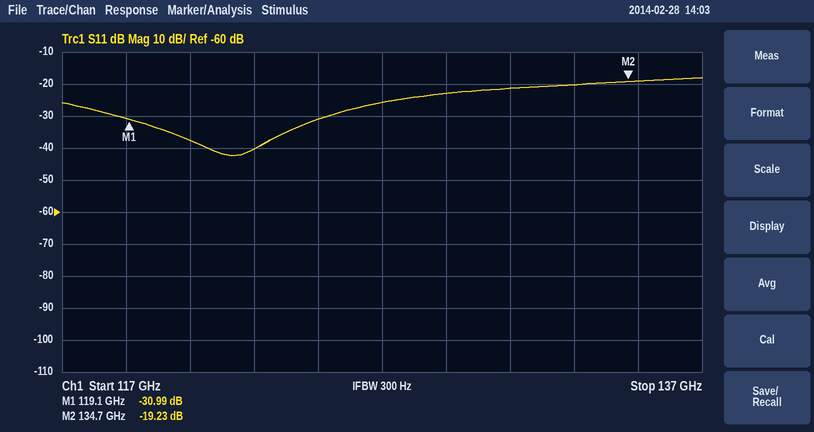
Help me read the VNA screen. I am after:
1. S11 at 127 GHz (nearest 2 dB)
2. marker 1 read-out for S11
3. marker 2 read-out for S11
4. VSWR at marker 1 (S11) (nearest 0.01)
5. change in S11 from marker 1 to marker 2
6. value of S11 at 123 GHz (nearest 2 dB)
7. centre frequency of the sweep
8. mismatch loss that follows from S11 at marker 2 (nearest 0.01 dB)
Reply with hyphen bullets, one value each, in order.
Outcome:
- -26 dB
- -30.99 dB
- -19.23 dB
- 1.06
- 11.76 dB
- -40 dB
- 127 GHz
- 0.05 dB
